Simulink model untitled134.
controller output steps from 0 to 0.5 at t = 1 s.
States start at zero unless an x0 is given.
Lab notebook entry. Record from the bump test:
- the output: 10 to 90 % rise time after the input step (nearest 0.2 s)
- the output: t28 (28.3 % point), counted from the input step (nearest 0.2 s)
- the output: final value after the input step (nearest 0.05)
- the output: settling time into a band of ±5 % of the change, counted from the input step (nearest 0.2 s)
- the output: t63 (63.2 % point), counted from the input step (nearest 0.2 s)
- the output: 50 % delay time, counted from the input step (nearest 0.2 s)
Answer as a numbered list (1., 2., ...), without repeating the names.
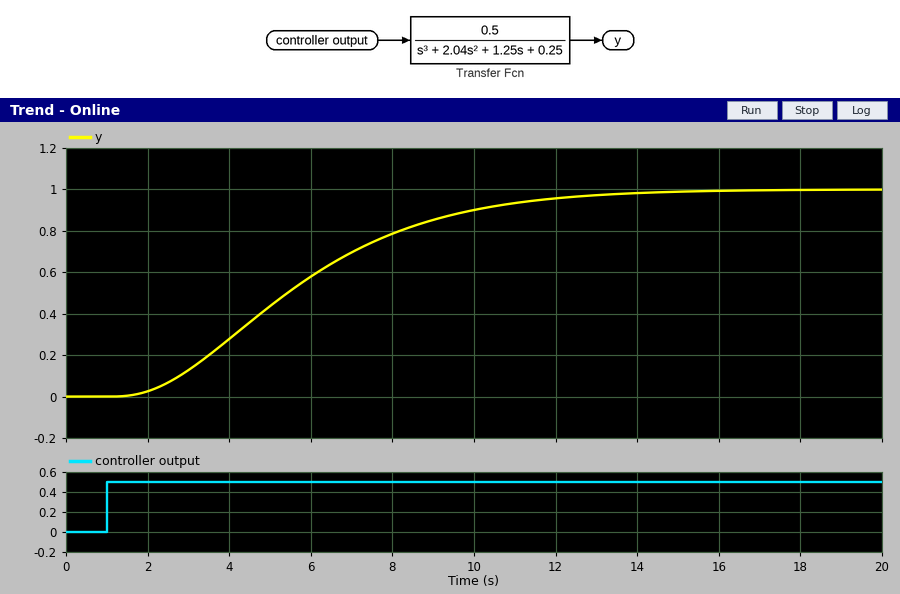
1. 7.2 s
2. 3.0 s
3. 1.00
4. 10.6 s
5. 5.4 s
6. 4.4 s
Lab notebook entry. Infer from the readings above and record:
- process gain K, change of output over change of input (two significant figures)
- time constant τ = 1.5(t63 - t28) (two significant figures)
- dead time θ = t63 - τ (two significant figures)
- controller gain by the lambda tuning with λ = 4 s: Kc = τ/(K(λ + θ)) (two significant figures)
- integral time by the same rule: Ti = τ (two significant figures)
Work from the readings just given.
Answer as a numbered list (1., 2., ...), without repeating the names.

1. 2.0
2. 3.6 s
3. 1.8 s
4. 0.31
5. 3.6 s
